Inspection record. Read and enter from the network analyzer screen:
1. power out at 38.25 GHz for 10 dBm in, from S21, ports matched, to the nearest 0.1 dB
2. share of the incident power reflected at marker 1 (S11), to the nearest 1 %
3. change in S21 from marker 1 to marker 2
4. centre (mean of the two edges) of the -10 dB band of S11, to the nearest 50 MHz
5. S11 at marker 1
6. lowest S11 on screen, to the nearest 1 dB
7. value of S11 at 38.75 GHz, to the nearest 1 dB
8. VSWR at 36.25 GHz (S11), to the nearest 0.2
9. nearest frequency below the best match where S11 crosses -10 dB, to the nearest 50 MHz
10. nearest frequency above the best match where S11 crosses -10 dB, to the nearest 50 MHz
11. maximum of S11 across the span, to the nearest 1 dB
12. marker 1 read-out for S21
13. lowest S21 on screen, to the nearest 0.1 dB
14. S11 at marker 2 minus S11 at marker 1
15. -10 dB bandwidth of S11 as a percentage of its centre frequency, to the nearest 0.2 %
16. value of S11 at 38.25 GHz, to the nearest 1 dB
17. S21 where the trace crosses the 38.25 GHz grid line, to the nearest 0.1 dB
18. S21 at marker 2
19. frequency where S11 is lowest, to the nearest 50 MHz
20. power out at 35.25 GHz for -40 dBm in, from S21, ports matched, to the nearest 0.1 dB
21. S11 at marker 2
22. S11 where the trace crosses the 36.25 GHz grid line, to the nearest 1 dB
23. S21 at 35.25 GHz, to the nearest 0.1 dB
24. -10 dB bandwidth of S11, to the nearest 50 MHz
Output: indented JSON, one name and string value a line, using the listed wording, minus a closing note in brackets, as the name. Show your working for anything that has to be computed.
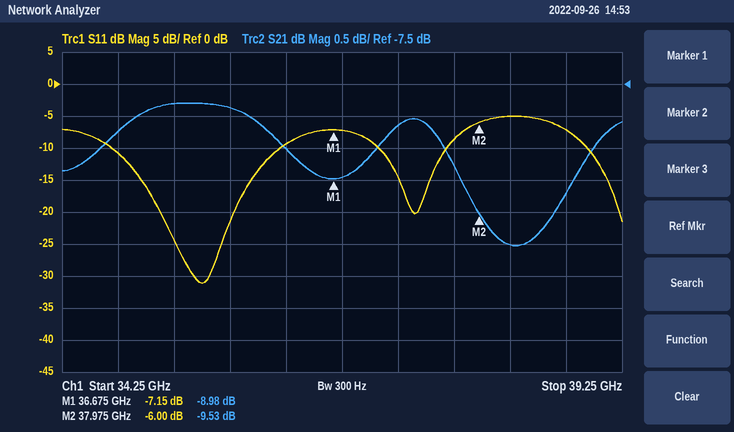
{
  "power out at 38.25 GHz for 10 dBm in, from S21, ports matched, to the nearest 0.1 dB": "10 dBm + (-10.0 dB) = 0.0 dBm",
  "share of the incident power reflected at marker 1 (S11), to the nearest 1 %": "10^(-7.15/10) ≈ 19 %",
  "change in S21 from marker 1 to marker 2": "-9.53 − (-8.98) = -0.55 dB",
  "centre (mean of the two edges) of the -10 dB band of S11, to the nearest 50 MHz": "35.45 GHz",
  "S11 at marker 1": "-7.15 dB",
  "lowest S11 on screen, to the nearest 1 dB": "-31 dB",
  "value of S11 at 38.75 GHz, to the nearest 1 dB": "-7 dB",
  "VSWR at 36.25 GHz (S11), to the nearest 0.2": "|Γ| = 10^(-9/20) = 0.3548; VSWR = (1 + 0.3548)/(1 − 0.3548) ≈ 2.10, so 2.0 to the nearest 0.2",
  "nearest frequency below the best match where S11 crosses -10 dB, to the nearest 50 MHz": "34.70 GHz",
  "nearest frequency above the best match where S11 crosses -10 dB, to the nearest 50 MHz": "36.20 GHz",
  "maximum of S11 across the span, to the nearest 1 dB": "-5 dB",
  "marker 1 read-out for S21": "-8.98 dB",
  "lowest S21 on screen, to the nearest 0.1 dB": "-10.0 dB",
  "S11 at marker 2 minus S11 at marker 1": "-6 − (-7.15) = 1.15 dB",
  "-10 dB bandwidth of S11 as a percentage of its centre frequency, to the nearest 0.2 %": "1.5 GHz / 35.45 GHz ≈ 4.2 %",
  "value of S11 at 38.25 GHz, to the nearest 1 dB": "-5 dB",
  "S21 where the trace crosses the 38.25 GHz grid line, to the nearest 0.1 dB": "-10.0 dB",
  "S21 at marker 2": "-9.53 dB",
  "frequency where S11 is lowest, to the nearest 50 MHz": "35.50 GHz",
  "power out at 35.25 GHz for -40 dBm in, from S21, ports matched, to the nearest 0.1 dB": "-40 dBm + (-7.8 dB) = -47.8 dBm",
  "S11 at marker 2": "-6.00 dB",
  "S11 where the trace crosses the 36.25 GHz grid line, to the nearest 1 dB": "-9 dB",
  "S21 at 35.25 GHz, to the nearest 0.1 dB": "-7.8 dB",
  "-10 dB bandwidth of S11, to the nearest 50 MHz": "36.20 GHz − 34.70 GHz = 1.50 GHz"
}
